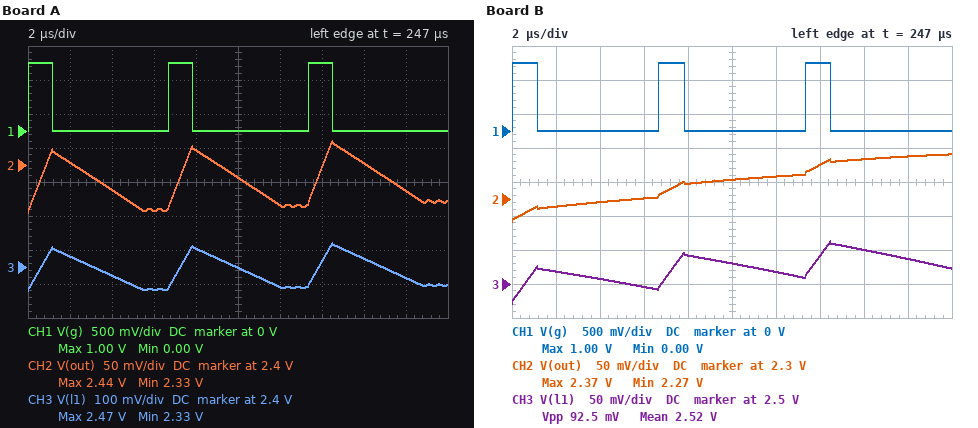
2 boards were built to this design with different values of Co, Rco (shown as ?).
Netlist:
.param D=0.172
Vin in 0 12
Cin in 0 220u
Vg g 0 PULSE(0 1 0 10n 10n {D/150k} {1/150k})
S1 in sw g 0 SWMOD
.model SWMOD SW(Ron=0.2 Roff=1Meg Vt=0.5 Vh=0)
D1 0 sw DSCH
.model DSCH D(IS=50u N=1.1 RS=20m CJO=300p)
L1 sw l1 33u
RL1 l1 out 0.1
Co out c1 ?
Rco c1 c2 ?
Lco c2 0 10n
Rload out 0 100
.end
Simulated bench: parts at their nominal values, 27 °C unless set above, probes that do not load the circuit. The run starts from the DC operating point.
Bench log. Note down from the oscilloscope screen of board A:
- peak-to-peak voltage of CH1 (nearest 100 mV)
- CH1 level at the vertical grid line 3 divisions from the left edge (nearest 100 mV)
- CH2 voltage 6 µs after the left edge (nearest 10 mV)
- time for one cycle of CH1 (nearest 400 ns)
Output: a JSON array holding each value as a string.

["1.0 V", "0 V", "2.33 V", "6.8 µs"]
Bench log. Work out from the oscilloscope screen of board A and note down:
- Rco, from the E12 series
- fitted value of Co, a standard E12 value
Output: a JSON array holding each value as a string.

["0.27 Ω", "120 µF"]
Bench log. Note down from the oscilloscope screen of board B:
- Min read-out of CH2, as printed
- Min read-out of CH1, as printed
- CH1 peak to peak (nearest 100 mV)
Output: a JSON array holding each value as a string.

["2.27 V", "0.00 V", "1.0 V"]
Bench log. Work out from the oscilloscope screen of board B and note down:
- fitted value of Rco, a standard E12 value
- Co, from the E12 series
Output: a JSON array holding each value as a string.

["0.039 Ω", "330 µF"]
